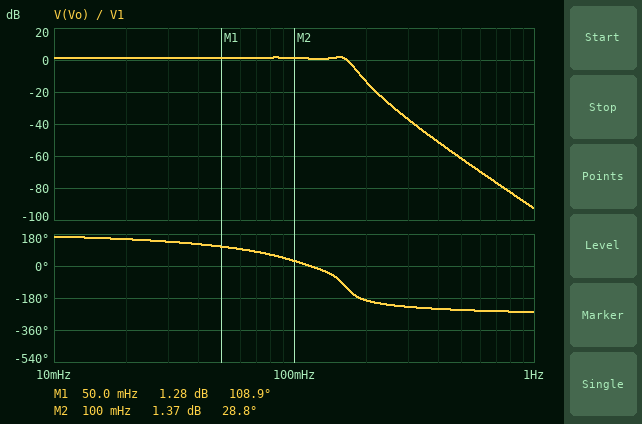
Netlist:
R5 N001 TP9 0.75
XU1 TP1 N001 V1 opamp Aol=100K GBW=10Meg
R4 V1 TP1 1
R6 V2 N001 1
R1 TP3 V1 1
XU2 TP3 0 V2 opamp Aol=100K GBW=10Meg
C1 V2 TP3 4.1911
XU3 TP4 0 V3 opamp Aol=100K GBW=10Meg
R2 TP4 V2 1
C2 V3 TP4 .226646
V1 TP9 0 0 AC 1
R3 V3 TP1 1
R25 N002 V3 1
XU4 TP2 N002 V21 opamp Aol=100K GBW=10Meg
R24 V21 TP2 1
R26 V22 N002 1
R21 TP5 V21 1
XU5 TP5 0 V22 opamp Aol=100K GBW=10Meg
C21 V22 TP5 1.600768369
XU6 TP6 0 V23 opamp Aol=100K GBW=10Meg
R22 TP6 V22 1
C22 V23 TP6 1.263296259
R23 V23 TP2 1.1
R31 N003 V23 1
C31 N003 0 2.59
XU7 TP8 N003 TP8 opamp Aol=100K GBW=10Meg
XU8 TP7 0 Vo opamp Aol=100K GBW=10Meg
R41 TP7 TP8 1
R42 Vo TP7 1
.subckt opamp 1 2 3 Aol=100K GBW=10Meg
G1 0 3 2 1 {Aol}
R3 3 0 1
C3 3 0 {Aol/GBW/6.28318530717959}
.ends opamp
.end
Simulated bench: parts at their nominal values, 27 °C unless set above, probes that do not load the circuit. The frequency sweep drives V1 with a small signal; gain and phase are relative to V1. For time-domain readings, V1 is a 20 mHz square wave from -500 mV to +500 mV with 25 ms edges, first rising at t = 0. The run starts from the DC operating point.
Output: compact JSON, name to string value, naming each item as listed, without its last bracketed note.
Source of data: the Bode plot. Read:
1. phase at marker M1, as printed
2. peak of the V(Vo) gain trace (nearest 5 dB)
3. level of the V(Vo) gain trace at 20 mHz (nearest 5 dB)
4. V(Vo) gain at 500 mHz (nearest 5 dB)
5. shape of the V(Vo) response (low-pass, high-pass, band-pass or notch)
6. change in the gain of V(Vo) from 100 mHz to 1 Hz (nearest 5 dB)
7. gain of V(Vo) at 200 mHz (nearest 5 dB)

{"phase at marker M1, as printed": "108.9 deg", "peak of the V(Vo) gain trace": "0 dB", "level of the V(Vo) gain trace at 20 mHz": "0 dB", "V(Vo) gain at 500 mHz": "-60 dB", "shape of the V(Vo) response": "low-pass", "change in the gain of V(Vo) from 100 mHz to 1 Hz": "-95 dB", "gain of V(Vo) at 200 mHz": "-15 dB"}
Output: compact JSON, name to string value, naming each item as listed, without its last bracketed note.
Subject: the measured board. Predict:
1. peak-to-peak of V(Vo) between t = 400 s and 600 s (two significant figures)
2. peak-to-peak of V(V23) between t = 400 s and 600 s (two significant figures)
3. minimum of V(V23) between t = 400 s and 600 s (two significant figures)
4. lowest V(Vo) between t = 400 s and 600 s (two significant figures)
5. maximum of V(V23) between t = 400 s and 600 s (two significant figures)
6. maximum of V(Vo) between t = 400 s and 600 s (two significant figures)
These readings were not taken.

{"peak-to-peak of V(Vo) between t = 400 s and 600 s": "1.5 V", "peak-to-peak of V(V23) between t = 400 s and 600 s": "2.7 V", "minimum of V(V23) between t = 400 s and 600 s": "-1.3 V", "lowest V(Vo) between t = 400 s and 600 s": "-760 mV", "maximum of V(V23) between t = 400 s and 600 s": "1.3 V", "maximum of V(Vo) between t = 400 s and 600 s": "760 mV"}
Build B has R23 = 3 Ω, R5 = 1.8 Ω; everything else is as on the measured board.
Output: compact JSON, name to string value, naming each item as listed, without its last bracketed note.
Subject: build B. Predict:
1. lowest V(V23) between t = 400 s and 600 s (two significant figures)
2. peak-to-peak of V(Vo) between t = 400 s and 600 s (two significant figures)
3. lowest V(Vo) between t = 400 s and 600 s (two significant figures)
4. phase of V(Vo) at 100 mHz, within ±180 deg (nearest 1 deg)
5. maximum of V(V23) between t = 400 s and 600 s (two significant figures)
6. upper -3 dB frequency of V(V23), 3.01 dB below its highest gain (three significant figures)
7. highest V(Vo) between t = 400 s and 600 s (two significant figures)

{"lowest V(V23) between t = 400 s and 600 s": "-950 mV", "peak-to-peak of V(Vo) between t = 400 s and 600 s": "1.7 V", "lowest V(Vo) between t = 400 s and 600 s": "-840 mV", "phase of V(Vo) at 100 mHz, within ±180 deg": "-26 deg", "maximum of V(V23) between t = 400 s and 600 s": "950 mV", "upper -3 dB frequency of V(V23), 3.01 dB below its highest gain": "85.1 mHz", "highest V(Vo) between t = 400 s and 600 s": "840 mV"}
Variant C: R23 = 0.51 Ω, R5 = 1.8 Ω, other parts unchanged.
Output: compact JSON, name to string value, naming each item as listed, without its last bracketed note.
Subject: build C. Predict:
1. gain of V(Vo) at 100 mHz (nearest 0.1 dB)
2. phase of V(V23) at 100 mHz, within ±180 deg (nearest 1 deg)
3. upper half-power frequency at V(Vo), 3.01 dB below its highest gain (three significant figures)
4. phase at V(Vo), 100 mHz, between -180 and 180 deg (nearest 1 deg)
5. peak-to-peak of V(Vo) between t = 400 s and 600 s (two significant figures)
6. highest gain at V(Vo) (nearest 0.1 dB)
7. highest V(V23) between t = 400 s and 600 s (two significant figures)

{"gain of V(Vo) at 100 mHz": "-5.8 dB", "phase of V(V23) at 100 mHz, within ±180 deg": "-62 deg", "upper half-power frequency at V(Vo), 3.01 dB below its highest gain": "173 mHz", "phase at V(Vo), 100 mHz, between -180 and 180 deg": "60 deg", "peak-to-peak of V(Vo) between t = 400 s and 600 s": "670 mV", "highest gain at V(Vo)": "-2.9 dB", "highest V(V23) between t = 400 s and 600 s": "650 mV"}
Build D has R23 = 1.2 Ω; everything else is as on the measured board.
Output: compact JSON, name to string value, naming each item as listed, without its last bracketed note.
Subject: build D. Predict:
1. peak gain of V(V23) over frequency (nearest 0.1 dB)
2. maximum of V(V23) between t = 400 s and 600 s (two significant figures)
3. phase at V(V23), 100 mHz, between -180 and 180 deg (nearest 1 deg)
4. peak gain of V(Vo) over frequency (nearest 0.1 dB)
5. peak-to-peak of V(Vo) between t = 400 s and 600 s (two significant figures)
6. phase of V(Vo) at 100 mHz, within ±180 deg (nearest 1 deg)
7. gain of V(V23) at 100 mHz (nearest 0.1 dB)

{"peak gain of V(V23) over frequency": "10.0 dB", "maximum of V(V23) between t = 400 s and 600 s": "1.4 V", "phase at V(V23), 100 mHz, between -180 and 180 deg": "-98 deg", "peak gain of V(Vo) over frequency": "2.0 dB", "peak-to-peak of V(Vo) between t = 400 s and 600 s": "1.6 V", "phase of V(Vo) at 100 mHz, within ±180 deg": "23 deg", "gain of V(V23) at 100 mHz": "7.1 dB"}
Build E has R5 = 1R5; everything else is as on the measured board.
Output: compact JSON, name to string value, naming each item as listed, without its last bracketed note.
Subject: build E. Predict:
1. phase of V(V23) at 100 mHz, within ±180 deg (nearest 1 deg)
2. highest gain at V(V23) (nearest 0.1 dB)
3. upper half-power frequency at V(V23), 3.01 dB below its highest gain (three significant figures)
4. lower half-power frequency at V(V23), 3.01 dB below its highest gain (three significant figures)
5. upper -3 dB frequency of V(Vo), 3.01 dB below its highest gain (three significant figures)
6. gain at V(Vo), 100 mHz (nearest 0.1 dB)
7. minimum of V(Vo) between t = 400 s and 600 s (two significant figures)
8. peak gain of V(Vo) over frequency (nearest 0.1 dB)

{"phase of V(V23) at 100 mHz, within ±180 deg": "-97 deg", "highest gain at V(V23)": "4.9 dB", "upper half-power frequency at V(V23), 3.01 dB below its highest gain": "172 mHz", "lower half-power frequency at V(V23), 3.01 dB below its highest gain": "69.9 mHz", "upper -3 dB frequency of V(Vo), 3.01 dB below its highest gain": "160 mHz", "gain at V(Vo), 100 mHz": "-1.9 dB", "minimum of V(Vo) between t = 400 s and 600 s": "-520 mV", "peak gain of V(Vo) over frequency": "-1.5 dB"}
